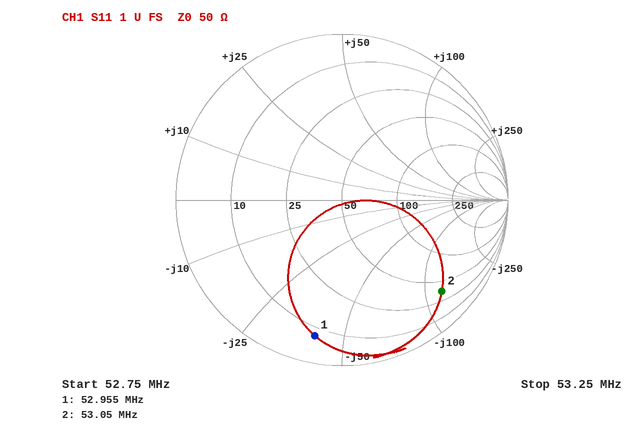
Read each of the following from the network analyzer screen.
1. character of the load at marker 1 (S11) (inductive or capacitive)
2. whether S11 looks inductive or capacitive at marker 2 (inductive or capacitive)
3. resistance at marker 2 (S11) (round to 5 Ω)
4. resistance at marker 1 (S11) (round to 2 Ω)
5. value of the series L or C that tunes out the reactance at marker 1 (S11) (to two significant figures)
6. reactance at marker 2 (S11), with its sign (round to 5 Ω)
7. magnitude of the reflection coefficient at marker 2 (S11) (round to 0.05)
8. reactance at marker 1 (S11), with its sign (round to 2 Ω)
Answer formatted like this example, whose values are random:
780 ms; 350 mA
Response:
capacitive; capacitive; 35 Ω; 8 Ω; 120 nH; -120 Ω; 0.80; -40 Ω
